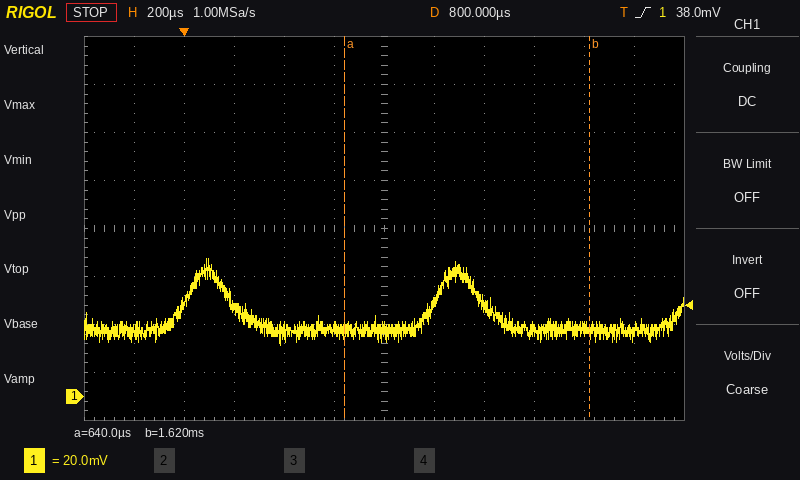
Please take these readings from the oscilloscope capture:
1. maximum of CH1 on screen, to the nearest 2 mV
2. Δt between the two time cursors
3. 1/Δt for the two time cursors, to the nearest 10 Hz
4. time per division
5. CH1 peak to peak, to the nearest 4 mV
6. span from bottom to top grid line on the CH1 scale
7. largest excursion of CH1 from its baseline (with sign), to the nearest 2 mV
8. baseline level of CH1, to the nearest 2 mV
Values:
58 mV
980 µs
1.02 kHz
200 µs
36 mV
160 mV
+30 mV
28 mV
